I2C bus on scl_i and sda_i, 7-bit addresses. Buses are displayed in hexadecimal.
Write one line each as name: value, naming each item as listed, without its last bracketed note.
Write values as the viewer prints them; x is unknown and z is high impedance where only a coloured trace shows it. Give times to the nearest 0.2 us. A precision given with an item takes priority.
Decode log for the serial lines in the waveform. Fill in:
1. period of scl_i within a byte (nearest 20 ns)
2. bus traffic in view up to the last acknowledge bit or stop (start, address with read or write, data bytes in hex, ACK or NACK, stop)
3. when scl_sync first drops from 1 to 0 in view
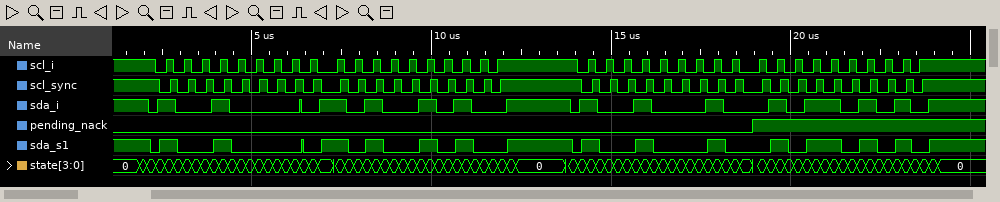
period of scl_i within a byte: 500 ns
bus traffic in view up to the last acknowledge bit or stop: start, address 48 write ACK, A5 ACK, stop, start, address 48 read ACK, 5A NACK, stop
when scl_sync first drops from 1 to 0 in view: 2.4 us
